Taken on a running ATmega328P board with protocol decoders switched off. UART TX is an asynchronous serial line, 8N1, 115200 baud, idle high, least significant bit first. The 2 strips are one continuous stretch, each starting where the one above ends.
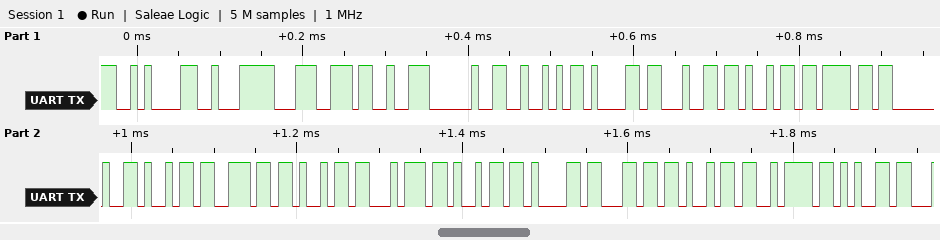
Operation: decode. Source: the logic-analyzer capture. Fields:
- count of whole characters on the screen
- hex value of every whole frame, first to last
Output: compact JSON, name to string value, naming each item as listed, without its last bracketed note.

{"count of whole characters on the screen": "21", "hex value of every whole frame, first to last": "0A E2 9C 93 20 52 61 64 69 6F 20 69 6E 69 74 69 61 6C 69 7A 65"}
